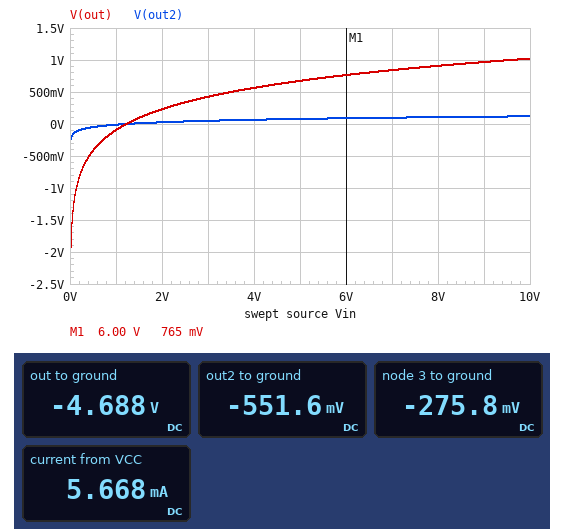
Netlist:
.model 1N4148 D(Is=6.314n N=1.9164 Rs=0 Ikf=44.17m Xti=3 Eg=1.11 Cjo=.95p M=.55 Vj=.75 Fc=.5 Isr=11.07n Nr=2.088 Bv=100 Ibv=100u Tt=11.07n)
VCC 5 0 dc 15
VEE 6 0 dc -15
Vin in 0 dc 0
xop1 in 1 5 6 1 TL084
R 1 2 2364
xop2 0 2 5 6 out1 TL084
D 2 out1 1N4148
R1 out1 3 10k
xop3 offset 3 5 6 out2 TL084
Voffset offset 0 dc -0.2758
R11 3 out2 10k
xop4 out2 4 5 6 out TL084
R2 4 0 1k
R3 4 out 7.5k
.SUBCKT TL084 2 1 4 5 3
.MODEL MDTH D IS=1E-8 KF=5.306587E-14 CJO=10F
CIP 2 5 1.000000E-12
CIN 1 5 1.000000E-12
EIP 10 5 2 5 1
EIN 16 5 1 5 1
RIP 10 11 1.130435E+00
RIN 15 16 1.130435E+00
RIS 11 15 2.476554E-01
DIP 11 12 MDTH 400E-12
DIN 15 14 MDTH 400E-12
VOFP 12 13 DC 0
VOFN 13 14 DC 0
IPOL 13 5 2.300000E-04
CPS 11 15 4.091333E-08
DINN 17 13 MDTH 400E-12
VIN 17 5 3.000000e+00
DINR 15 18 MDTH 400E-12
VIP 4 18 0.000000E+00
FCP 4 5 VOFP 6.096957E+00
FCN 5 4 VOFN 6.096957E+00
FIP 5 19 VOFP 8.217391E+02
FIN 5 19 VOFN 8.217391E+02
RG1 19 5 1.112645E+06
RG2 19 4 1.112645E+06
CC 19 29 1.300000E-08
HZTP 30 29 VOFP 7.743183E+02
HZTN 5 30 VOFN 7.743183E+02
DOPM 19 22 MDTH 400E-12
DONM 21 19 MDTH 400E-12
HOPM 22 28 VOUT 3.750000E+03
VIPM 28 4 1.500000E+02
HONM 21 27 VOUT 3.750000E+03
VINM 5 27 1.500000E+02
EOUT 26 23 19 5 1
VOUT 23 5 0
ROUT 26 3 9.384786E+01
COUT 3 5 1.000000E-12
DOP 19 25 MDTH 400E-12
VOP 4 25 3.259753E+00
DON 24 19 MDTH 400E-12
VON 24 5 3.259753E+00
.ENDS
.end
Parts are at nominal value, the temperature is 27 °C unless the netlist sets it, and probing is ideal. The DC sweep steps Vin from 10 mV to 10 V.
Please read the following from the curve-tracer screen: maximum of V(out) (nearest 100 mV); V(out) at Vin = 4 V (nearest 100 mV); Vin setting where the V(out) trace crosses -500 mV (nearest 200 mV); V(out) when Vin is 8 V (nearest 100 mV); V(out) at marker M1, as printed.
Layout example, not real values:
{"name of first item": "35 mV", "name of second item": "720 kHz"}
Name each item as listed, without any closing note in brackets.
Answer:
{"maximum of V(out)": "1.0 V", "V(out) at Vin = 4 V": "600 mV", "Vin setting where the V(out) trace crosses -500 mV": "400 mV", "V(out) when Vin is 8 V": "900 mV", "V(out) at marker M1, as printed": "765 mV"}
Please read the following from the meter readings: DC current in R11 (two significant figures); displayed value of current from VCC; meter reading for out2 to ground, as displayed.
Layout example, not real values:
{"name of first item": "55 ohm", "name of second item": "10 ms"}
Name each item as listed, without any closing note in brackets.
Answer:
{"DC current in R11": "28 µA", "displayed value of current from VCC": "5.668 mA", "meter reading for out2 to ground, as displayed": "-551.6 mV"}
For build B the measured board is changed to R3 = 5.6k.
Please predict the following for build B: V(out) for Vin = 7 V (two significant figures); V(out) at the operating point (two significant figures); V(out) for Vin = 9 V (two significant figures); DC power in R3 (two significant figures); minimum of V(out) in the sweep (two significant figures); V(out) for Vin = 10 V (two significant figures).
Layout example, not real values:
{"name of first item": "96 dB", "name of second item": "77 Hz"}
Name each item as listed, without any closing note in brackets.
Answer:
{"V(out) for Vin = 7 V": "650 mV", "V(out) at the operating point": "-3.6 V", "V(out) for Vin = 9 V": "750 mV", "DC power in R3": "1.7 mW", "minimum of V(out) in the sweep": "-1.7 V", "V(out) for Vin = 10 V": "790 mV"}
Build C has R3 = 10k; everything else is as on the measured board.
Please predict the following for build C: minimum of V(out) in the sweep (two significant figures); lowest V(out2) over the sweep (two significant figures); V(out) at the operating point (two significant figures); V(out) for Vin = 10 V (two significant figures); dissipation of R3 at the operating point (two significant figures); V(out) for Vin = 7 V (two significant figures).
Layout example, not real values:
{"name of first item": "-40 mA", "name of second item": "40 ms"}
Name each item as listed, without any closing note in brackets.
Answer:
{"minimum of V(out) in the sweep": "-2.8 V", "lowest V(out2) over the sweep": "-260 mV", "V(out) at the operating point": "-6.1 V", "V(out) for Vin = 10 V": "1.3 V", "dissipation of R3 at the operating point": "3.0 mW", "V(out) for Vin = 7 V": "1.1 V"}
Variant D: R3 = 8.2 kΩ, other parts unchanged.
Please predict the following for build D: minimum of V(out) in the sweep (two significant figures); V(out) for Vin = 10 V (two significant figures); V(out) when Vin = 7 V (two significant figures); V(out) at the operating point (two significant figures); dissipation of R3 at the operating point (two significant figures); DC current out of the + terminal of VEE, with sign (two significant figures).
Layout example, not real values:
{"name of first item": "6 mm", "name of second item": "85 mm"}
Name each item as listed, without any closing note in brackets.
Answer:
{"minimum of V(out) in the sweep": "-2.4 V", "V(out) for Vin = 10 V": "1.1 V", "V(out) when Vin = 7 V": "910 mV", "V(out) at the operating point": "-5.1 V", "dissipation of R3 at the operating point": "2.5 mW", "DC current out of the + terminal of VEE, with sign": "-6.2 mA"}
